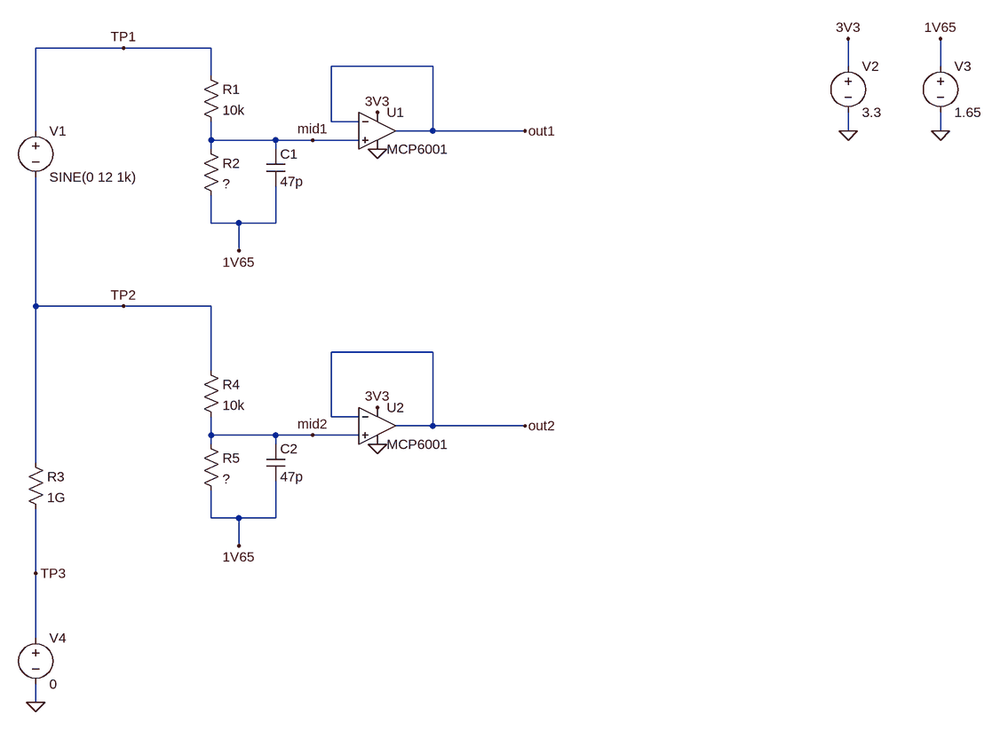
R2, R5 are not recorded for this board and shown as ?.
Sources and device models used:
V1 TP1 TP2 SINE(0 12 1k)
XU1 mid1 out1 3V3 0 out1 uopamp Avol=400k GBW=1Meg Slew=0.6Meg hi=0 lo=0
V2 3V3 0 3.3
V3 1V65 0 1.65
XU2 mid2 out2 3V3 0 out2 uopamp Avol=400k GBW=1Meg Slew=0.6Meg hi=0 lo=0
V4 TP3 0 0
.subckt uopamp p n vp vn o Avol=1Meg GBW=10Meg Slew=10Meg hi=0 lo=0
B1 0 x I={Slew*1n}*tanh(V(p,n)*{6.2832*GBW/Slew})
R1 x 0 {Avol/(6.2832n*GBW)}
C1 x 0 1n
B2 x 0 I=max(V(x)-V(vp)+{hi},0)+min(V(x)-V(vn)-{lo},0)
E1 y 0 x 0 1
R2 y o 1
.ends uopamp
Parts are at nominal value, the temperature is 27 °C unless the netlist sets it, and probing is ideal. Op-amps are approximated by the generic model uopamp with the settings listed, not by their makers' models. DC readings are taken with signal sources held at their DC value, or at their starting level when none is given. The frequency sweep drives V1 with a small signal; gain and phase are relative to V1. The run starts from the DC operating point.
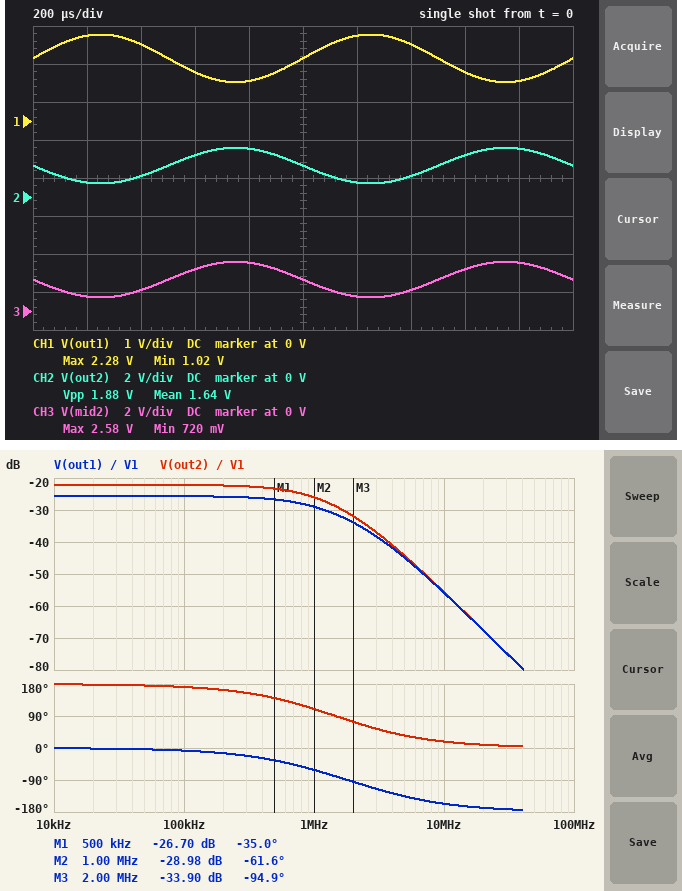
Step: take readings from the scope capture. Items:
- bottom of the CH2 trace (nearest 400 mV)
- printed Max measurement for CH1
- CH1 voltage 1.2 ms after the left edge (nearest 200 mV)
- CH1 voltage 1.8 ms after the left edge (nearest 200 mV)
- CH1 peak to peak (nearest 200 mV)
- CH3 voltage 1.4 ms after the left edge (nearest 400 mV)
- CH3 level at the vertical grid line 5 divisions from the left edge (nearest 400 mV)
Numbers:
800 mV
2.28 V
2.2 V
1.0 V
1.2 V
1.2 V
1.6 V
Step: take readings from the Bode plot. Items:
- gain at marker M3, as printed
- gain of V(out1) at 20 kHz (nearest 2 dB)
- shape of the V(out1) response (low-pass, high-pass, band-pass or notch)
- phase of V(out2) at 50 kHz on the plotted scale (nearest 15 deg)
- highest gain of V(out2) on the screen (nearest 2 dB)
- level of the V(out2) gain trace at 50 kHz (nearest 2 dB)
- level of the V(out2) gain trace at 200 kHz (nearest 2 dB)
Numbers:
-33.90 dB
-26 dB
low-pass
180 deg
-22 dB
-22 dB
-22 dB
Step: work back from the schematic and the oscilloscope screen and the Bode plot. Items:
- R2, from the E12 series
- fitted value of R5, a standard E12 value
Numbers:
1.2 kΩ
1.8 kΩ
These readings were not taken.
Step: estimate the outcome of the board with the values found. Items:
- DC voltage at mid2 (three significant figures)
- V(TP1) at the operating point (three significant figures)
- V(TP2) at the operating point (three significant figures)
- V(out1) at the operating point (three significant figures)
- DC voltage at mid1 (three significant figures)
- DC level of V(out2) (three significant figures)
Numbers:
1.65 V
1.65 V
1.65 V
1.65 V
1.65 V
1.65 V
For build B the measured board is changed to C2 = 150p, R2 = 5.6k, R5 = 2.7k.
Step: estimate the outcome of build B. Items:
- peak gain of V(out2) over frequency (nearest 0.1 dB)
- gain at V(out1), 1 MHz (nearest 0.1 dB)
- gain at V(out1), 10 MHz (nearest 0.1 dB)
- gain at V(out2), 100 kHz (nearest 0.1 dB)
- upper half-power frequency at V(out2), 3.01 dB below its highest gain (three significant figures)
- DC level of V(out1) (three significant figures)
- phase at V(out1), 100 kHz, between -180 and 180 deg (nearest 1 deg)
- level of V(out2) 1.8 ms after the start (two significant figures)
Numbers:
-20.4 dB
-20.7 dB
-55.5 dB
-20.6 dB
416 kHz
1.65 V
-12 deg
2.7 V
